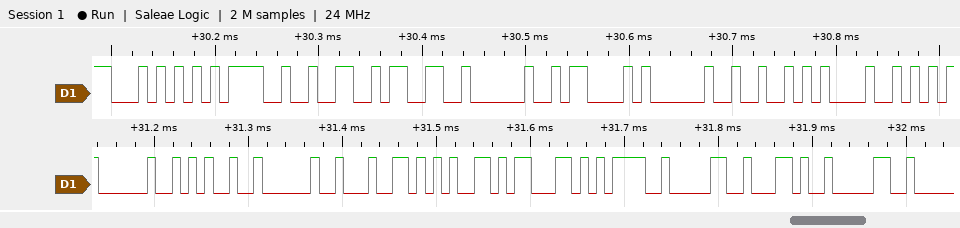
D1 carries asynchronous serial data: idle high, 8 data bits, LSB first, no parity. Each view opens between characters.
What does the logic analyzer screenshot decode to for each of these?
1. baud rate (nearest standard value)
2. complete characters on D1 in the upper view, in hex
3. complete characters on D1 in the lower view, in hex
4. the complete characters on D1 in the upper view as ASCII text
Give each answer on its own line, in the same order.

115200 baud
54, 3D, 32, 33, 20, 43, 20, 52, 48
20, 25, 20, 64, 65, 63, 3D, 30, 2C, 30
"T=23 C RH"
